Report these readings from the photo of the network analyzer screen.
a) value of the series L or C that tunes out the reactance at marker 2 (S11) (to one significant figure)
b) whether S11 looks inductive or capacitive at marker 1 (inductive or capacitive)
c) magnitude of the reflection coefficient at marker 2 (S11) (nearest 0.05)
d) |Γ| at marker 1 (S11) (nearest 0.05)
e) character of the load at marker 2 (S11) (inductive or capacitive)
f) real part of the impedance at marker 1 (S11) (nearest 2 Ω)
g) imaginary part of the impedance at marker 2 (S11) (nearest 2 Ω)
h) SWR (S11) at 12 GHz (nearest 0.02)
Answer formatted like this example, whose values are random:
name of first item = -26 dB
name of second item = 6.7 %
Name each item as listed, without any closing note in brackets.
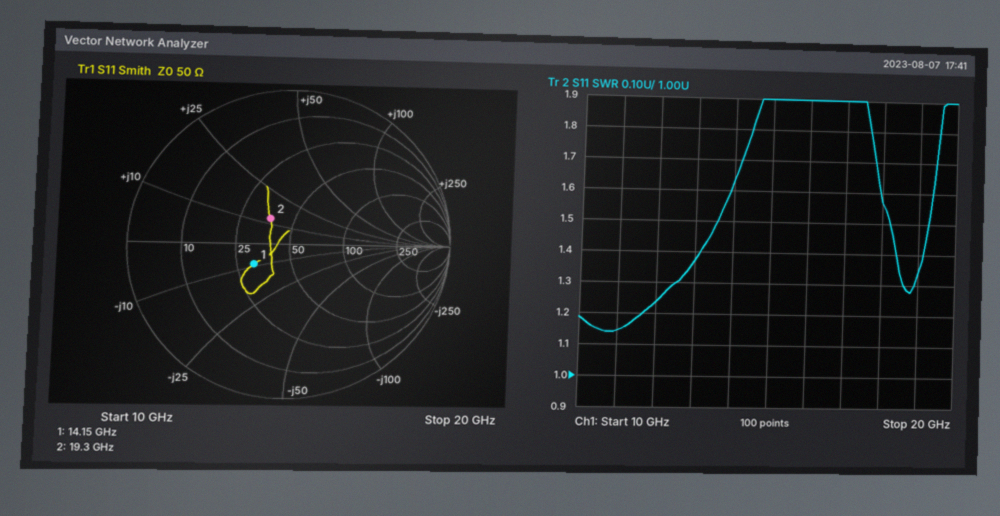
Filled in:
value of the series L or C that tunes out the reactance at marker 2 (S11) = 700 fF
whether S11 looks inductive or capacitive at marker 1 = capacitive
magnitude of the reflection coefficient at marker 2 (S11) = 0.20
|Γ| at marker 1 (S11) = 0.25
character of the load at marker 2 (S11) = inductive
real part of the impedance at marker 1 (S11) = 32 Ω
imaginary part of the impedance at marker 2 (S11) = +12 Ω
SWR (S11) at 12 GHz = 1.24
